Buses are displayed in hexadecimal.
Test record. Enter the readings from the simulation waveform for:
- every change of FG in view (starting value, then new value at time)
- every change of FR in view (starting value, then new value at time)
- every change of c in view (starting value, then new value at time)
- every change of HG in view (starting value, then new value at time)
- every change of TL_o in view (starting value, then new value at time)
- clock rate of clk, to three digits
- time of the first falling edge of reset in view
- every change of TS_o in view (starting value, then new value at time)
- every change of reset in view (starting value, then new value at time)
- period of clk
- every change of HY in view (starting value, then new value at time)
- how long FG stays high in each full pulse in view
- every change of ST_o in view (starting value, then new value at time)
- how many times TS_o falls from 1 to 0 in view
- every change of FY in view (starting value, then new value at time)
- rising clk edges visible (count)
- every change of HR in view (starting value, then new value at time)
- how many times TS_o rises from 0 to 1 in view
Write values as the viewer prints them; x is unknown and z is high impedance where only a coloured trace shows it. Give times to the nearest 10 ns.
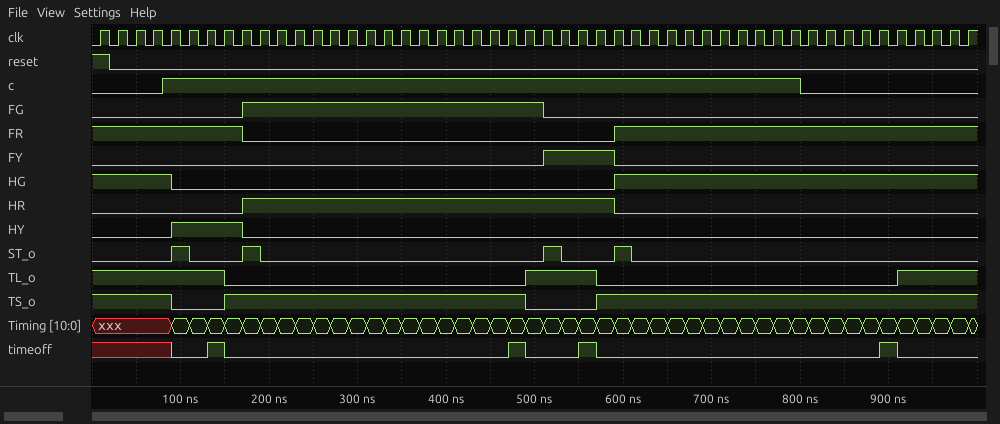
0, 1 at 170 ns, 0 at 510 ns
1, 0 at 170 ns, 1 at 590 ns
0, 1 at 80 ns, 0 at 800 ns
1, 0 at 90 ns, 1 at 590 ns
1, 0 at 150 ns, 1 at 490 ns, 0 at 570 ns, 1 at 910 ns
50.0 MHz
20 ns
1, 0 at 90 ns, 1 at 150 ns, 0 at 490 ns, 1 at 570 ns
1, 0 at 20 ns
20 ns
0, 1 at 90 ns, 0 at 170 ns
340 ns
0, 1 at 90 ns, 0 at 110 ns, 1 at 170 ns, 0 at 190 ns, 1 at 510 ns, 0 at 530 ns, 1 at 590 ns, 0 at 610 ns
2
0, 1 at 510 ns, 0 at 590 ns
50
0, 1 at 170 ns, 0 at 590 ns
2
